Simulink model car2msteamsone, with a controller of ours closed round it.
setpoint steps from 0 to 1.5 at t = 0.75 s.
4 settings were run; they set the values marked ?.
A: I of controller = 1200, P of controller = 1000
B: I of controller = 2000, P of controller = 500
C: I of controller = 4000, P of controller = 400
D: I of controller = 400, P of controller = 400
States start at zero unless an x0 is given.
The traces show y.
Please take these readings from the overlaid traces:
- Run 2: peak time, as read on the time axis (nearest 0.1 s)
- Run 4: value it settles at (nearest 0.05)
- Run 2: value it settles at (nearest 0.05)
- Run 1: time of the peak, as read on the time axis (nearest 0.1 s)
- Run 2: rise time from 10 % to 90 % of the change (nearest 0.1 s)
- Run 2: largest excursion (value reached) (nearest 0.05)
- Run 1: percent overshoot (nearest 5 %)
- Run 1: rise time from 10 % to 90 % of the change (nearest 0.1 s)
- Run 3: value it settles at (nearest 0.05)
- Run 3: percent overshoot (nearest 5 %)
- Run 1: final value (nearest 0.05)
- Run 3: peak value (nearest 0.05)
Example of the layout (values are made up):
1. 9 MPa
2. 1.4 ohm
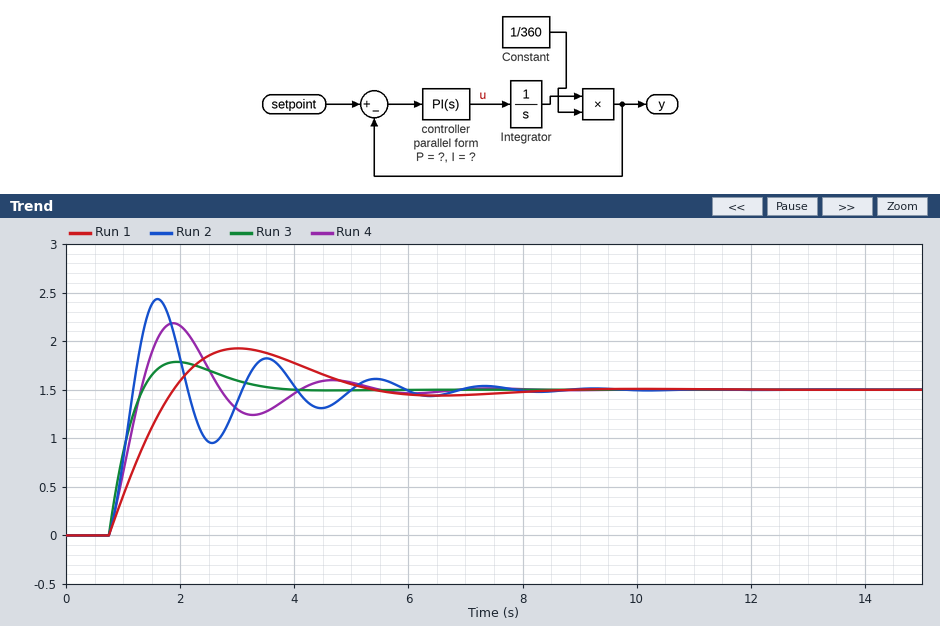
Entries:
1. 1.6 s
2. 1.50
3. 1.50
4. 3.0 s
5. 0.3 s
6. 2.45
7. 30 %
8. 0.9 s
9. 1.50
10. 20 %
11. 1.50
12. 1.80
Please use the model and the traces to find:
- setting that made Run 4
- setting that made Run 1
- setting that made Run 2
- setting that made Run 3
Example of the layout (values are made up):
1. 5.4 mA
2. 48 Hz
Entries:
1. B
2. D
3. C
4. A
